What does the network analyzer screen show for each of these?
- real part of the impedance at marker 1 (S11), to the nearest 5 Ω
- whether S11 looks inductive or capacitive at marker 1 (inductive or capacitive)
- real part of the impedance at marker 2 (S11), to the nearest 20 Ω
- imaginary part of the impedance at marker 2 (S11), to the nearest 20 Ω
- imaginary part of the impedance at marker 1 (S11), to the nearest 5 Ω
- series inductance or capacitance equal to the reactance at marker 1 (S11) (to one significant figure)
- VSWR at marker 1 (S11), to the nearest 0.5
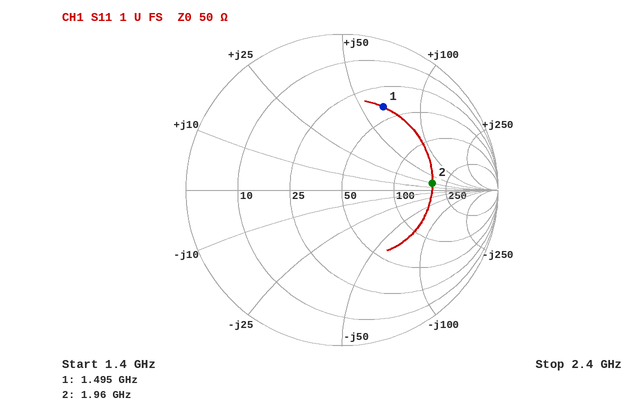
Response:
40 Ω
inductive
180 Ω
+20 Ω
+65 Ω
7 nH
4.0
